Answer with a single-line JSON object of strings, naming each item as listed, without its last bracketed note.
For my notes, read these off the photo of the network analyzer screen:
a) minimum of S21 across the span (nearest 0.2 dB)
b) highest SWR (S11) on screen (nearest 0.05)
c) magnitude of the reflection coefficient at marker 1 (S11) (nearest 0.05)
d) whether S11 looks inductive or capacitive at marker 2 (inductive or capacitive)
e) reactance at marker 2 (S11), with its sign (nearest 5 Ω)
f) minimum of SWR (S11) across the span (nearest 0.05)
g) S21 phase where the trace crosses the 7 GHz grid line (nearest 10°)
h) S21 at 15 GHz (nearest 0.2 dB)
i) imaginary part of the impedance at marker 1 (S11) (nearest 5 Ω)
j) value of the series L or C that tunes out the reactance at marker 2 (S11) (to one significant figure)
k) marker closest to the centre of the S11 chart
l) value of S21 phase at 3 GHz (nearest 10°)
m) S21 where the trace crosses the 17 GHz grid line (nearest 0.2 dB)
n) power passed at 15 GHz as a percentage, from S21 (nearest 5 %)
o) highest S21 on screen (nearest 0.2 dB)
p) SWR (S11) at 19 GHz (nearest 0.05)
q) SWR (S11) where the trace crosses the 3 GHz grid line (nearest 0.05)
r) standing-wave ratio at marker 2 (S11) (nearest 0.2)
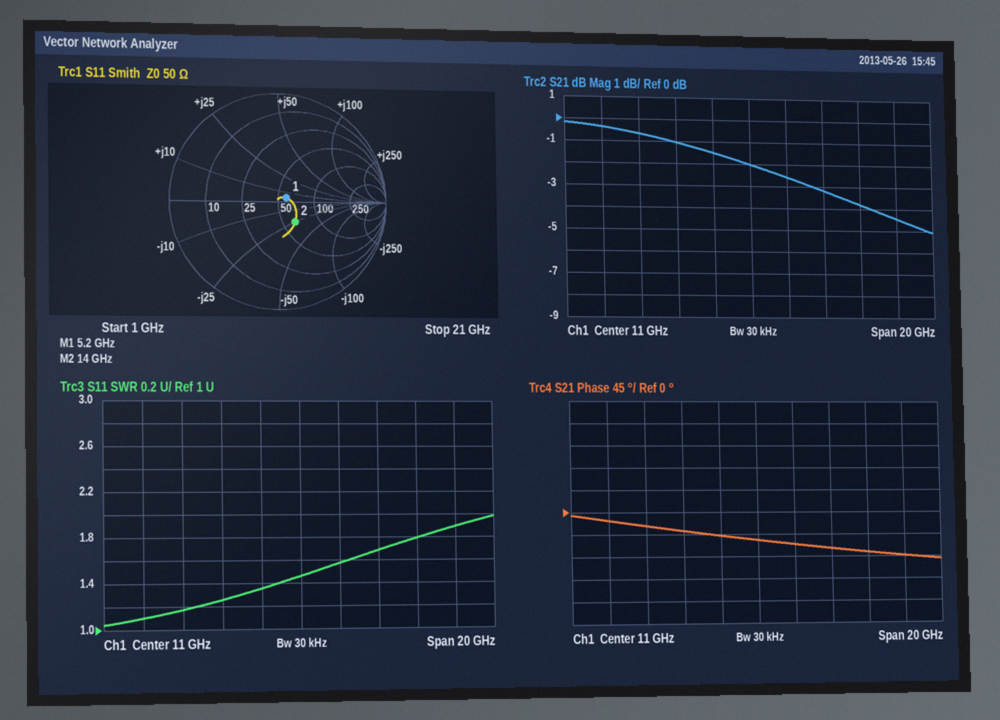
{"minimum of S21 across the span": "-5.0 dB", "highest SWR (S11) on screen": "2.00", "magnitude of the reflection coefficient at marker 1 (S11)": "0.10", "whether S11 looks inductive or capacitive at marker 2": "capacitive", "reactance at marker 2 (S11), with its sign": "-25 Ω", "minimum of SWR (S11) across the span": "1.05", "S21 phase where the trace crosses the 7 GHz grid line": "-40°", "S21 at 15 GHz": "-3.2 dB", "imaginary part of the impedance at marker 1 (S11)": "+5 Ω", "value of the series L or C that tunes out the reactance at marker 2 (S11)": "300 pH", "marker closest to the centre of the S11 chart": "marker 1", "value of S21 phase at 3 GHz": "-20°", "S21 where the trace crosses the 17 GHz grid line": "-3.8 dB", "power passed at 15 GHz as a percentage, from S21": "50 %", "highest S21 on screen": "-0.2 dB", "SWR (S11) at 19 GHz": "1.90", "SWR (S11) where the trace crosses the 3 GHz grid line": "1.10", "standing-wave ratio at marker 2 (S11)": "1.6"}
